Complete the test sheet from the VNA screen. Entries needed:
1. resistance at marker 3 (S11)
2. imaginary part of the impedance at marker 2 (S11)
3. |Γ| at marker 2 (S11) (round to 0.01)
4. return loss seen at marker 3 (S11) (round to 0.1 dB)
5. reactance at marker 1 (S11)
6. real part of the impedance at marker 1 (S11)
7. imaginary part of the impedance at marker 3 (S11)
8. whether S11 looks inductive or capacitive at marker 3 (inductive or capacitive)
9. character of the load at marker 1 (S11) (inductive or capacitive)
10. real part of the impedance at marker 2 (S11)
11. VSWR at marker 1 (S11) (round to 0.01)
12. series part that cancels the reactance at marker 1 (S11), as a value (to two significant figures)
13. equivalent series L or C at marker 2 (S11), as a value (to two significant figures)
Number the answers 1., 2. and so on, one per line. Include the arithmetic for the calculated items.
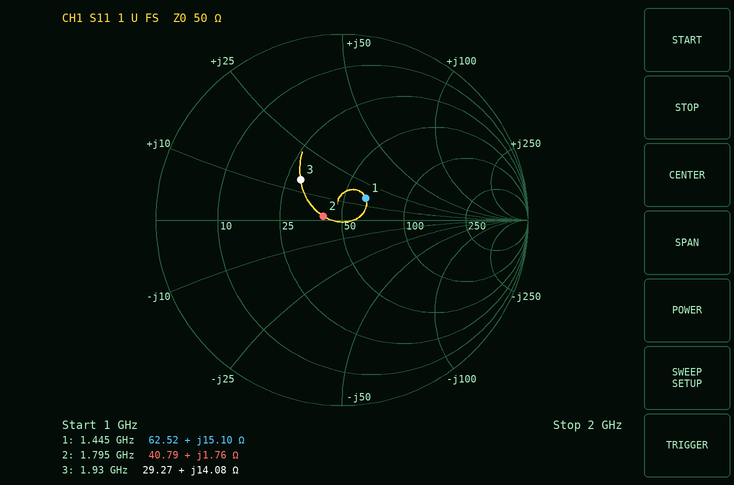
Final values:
1. 29.27 Ω
2. +1.76 Ω
3. 0.10
4. 10.1 dB
5. +15.10 Ω
6. 62.52 Ω
7. +14.08 Ω
8. inductive
9. inductive
10. 40.79 Ω
11. 1.42
12. C = 1/(2π × 1.445 GHz × 15.1 Ω) ≈ 7.3 pF
13. L = 1.76 Ω/(2π × 1.795 GHz) ≈ 156 pH, so 160 pH to two significant figures
